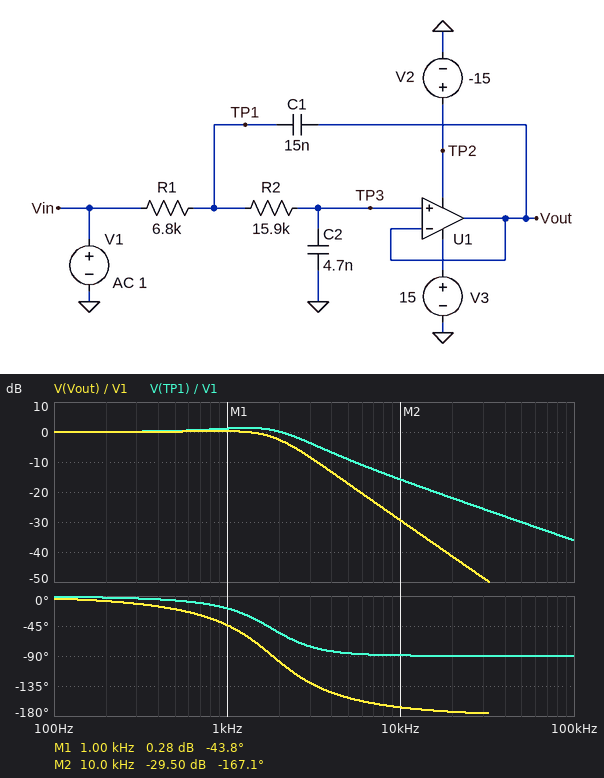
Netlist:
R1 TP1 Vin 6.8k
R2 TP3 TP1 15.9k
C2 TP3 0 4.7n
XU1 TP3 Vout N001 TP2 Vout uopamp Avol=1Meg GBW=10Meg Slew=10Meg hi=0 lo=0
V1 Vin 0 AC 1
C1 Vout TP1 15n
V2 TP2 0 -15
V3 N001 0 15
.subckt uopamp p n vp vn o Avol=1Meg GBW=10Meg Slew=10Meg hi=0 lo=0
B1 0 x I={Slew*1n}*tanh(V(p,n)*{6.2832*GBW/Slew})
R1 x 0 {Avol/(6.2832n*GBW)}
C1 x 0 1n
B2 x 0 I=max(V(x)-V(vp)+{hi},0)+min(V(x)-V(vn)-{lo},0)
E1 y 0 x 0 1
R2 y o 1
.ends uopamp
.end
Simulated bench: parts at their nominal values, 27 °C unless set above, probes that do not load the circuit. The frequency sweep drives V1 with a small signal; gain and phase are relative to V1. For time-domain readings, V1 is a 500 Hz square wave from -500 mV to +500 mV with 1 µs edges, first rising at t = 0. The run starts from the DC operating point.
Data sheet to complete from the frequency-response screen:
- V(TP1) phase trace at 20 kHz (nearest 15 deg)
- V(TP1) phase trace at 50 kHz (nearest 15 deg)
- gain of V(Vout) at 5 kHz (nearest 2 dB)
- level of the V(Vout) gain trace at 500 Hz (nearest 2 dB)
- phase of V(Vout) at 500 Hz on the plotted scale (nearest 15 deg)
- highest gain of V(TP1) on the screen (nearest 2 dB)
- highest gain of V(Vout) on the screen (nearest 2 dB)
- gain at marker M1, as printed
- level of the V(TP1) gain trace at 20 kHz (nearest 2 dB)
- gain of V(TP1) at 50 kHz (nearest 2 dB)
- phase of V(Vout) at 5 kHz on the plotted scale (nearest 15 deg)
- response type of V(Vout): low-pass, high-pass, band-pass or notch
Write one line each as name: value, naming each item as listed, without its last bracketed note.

V(TP1) phase trace at 20 kHz: -90 deg
V(TP1) phase trace at 50 kHz: -90 deg
gain of V(Vout) at 5 kHz: -18 dB
level of the V(Vout) gain trace at 500 Hz: 0 dB
phase of V(Vout) at 500 Hz on the plotted scale: -15 deg
highest gain of V(TP1) on the screen: 2 dB
highest gain of V(Vout) on the screen: 0 dB
gain at marker M1, as printed: 0.28 dB
level of the V(TP1) gain trace at 20 kHz: -22 dB
gain of V(TP1) at 50 kHz: -30 dB
phase of V(Vout) at 5 kHz on the plotted scale: -150 deg
response type of V(Vout): low-pass, high-pass, band-pass or notch: low-pass
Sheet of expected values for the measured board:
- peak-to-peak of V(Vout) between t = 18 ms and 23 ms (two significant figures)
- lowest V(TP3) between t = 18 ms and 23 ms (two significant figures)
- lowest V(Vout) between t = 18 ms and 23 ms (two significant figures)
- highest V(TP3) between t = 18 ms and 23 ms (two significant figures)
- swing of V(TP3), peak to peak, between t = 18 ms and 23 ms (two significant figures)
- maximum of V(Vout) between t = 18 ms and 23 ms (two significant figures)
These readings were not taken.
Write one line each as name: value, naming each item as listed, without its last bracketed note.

peak-to-peak of V(Vout) between t = 18 ms and 23 ms: 1.2 V
lowest V(TP3) between t = 18 ms and 23 ms: -590 mV
lowest V(Vout) between t = 18 ms and 23 ms: -590 mV
highest V(TP3) between t = 18 ms and 23 ms: 590 mV
swing of V(TP3), peak to peak, between t = 18 ms and 23 ms: 1.2 V
maximum of V(Vout) between t = 18 ms and 23 ms: 590 mV
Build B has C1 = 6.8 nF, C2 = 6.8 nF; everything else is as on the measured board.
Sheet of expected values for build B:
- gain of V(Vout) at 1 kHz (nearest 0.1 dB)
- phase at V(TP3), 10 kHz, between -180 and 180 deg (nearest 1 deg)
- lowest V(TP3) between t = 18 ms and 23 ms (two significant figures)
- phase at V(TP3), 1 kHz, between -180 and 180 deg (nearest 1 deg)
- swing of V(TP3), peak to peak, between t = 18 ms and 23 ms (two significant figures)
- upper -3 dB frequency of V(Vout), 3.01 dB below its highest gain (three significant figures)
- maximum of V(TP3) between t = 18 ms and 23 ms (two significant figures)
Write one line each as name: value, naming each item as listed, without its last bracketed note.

gain of V(Vout) at 1 kHz: -2.0 dB
phase at V(TP3), 10 kHz, between -180 and 180 deg: -153 deg
lowest V(TP3) between t = 18 ms and 23 ms: -500 mV
phase at V(TP3), 1 kHz, between -180 and 180 deg: -50 deg
swing of V(TP3), peak to peak, between t = 18 ms and 23 ms: 1.0 V
upper -3 dB frequency of V(Vout), 3.01 dB below its highest gain: 1.28 kHz
maximum of V(TP3) between t = 18 ms and 23 ms: 500 mV
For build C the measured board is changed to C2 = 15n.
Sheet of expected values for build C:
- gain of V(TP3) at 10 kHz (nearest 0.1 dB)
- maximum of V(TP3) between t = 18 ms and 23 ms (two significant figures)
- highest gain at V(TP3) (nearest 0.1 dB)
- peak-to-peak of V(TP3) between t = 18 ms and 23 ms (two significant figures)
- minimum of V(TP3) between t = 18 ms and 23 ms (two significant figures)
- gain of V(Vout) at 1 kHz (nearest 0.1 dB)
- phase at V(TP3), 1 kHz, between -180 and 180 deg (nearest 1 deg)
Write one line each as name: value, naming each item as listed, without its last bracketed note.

gain of V(TP3) at 10 kHz: -39.8 dB
maximum of V(TP3) between t = 18 ms and 23 ms: 470 mV
highest gain at V(TP3): 0 dB
peak-to-peak of V(TP3) between t = 18 ms and 23 ms: 950 mV
minimum of V(TP3) between t = 18 ms and 23 ms: -470 mV
gain of V(Vout) at 1 kHz: -6.6 dB
phase at V(TP3), 1 kHz, between -180 and 180 deg: -89 deg
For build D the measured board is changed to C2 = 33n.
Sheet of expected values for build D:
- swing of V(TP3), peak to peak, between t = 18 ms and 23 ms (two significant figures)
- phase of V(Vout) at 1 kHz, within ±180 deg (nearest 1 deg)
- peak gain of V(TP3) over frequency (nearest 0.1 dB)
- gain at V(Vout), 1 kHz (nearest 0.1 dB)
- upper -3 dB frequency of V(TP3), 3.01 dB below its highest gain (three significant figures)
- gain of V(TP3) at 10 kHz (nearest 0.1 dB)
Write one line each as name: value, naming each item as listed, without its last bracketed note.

swing of V(TP3), peak to peak, between t = 18 ms and 23 ms: 590 mV
phase of V(Vout) at 1 kHz, within ±180 deg: -103 deg
peak gain of V(TP3) over frequency: 0 dB
gain at V(Vout), 1 kHz: -13.7 dB
upper -3 dB frequency of V(TP3), 3.01 dB below its highest gain: 235 Hz
gain of V(TP3) at 10 kHz: -46.7 dB
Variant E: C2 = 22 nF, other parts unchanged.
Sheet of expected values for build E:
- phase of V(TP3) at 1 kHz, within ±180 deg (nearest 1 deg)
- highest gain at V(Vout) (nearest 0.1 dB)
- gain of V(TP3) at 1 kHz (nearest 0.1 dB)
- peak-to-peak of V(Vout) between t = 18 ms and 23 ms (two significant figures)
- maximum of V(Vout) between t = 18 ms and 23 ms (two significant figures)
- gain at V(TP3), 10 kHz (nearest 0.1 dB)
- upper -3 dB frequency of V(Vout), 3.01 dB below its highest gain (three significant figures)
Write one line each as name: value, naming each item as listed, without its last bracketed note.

phase of V(TP3) at 1 kHz, within ±180 deg: -97 deg
highest gain at V(Vout): 0 dB
gain of V(TP3) at 1 kHz: -10.0 dB
peak-to-peak of V(Vout) between t = 18 ms and 23 ms: 800 mV
maximum of V(Vout) between t = 18 ms and 23 ms: 400 mV
gain at V(TP3), 10 kHz: -43.1 dB
upper -3 dB frequency of V(Vout), 3.01 dB below its highest gain: 370 Hz
